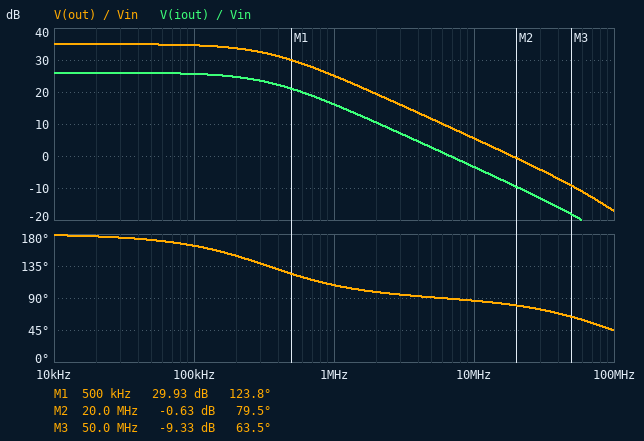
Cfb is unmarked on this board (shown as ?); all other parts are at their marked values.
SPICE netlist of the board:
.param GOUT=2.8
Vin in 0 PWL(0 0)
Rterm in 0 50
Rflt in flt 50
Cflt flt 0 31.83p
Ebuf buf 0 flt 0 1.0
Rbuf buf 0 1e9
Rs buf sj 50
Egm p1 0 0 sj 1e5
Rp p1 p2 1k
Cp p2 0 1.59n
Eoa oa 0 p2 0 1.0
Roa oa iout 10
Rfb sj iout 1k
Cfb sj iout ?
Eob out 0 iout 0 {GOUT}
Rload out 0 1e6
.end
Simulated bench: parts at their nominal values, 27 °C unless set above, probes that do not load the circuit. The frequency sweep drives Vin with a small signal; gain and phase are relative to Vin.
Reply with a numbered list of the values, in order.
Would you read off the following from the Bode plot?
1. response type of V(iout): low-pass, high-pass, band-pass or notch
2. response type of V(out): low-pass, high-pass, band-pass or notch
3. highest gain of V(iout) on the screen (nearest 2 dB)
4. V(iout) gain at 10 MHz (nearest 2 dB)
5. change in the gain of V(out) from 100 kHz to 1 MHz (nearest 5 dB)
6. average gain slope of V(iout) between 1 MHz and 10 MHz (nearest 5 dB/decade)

1. low-pass
2. low-pass
3. 26 dB
4. -4 dB
5. -10 dB
6. -20 dB/decade
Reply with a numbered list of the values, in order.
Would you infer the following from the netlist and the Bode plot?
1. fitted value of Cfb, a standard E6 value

1. 470 pF
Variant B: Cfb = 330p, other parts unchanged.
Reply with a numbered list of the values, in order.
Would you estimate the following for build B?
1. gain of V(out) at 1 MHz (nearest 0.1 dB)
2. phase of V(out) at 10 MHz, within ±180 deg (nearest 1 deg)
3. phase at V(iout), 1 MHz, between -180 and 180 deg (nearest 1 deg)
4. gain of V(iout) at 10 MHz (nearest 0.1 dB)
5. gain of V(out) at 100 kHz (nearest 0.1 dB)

1. 27.7 dB
2. 87 deg
3. 115 deg
4. -0.4 dB
5. 34.8 dB
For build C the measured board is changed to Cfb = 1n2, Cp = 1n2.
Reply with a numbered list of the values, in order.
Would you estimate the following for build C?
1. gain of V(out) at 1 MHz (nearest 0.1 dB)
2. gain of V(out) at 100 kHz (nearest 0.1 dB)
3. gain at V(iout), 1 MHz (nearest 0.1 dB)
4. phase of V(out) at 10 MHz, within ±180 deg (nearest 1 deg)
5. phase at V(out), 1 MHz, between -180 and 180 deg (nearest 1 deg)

1. 17.3 dB
2. 33.0 dB
3. 8.4 dB
4. 85 deg
5. 97 deg
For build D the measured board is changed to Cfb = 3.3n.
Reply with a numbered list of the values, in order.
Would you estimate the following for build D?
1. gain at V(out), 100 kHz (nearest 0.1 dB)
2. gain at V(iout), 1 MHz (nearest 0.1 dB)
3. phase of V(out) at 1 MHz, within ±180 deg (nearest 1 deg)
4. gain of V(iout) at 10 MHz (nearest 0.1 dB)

1. 27.7 dB
2. -0.3 dB
3. 92 deg
4. -20.3 dB
